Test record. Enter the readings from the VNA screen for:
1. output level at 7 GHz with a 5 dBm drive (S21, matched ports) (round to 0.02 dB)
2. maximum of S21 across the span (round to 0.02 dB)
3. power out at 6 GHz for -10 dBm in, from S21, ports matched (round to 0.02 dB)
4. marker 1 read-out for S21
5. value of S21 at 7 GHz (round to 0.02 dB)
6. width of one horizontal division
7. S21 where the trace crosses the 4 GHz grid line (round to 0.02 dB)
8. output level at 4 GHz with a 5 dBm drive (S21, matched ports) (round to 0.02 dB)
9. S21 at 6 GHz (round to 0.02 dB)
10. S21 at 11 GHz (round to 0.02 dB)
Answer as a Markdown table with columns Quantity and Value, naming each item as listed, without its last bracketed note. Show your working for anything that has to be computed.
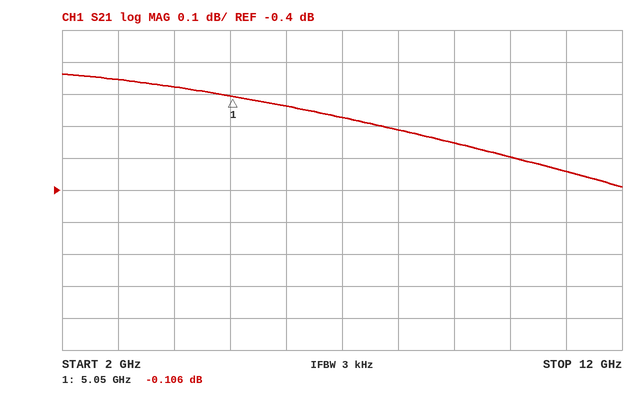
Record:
| Quantity | Value |
|---|---|
| output level at 7 GHz with a 5 dBm drive (S21, matched ports) | 5 dBm + (-0.18 dB) = 4.82 dBm |
| maximum of S21 across the span | -0.04 dB |
| power out at 6 GHz for -10 dBm in, from S21, ports matched | -10 dBm + (-0.14 dB) = -10.14 dBm |
| marker 1 read-out for S21 | -0.106 dB |
| value of S21 at 7 GHz | -0.18 dB |
| width of one horizontal division | 1 GHz |
| S21 where the trace crosses the 4 GHz grid line | -0.08 dB |
| output level at 4 GHz with a 5 dBm drive (S21, matched ports) | 5 dBm + (-0.08 dB) = 4.92 dBm |
| S21 at 6 GHz | -0.14 dB |
| S21 at 11 GHz | -0.34 dB |
